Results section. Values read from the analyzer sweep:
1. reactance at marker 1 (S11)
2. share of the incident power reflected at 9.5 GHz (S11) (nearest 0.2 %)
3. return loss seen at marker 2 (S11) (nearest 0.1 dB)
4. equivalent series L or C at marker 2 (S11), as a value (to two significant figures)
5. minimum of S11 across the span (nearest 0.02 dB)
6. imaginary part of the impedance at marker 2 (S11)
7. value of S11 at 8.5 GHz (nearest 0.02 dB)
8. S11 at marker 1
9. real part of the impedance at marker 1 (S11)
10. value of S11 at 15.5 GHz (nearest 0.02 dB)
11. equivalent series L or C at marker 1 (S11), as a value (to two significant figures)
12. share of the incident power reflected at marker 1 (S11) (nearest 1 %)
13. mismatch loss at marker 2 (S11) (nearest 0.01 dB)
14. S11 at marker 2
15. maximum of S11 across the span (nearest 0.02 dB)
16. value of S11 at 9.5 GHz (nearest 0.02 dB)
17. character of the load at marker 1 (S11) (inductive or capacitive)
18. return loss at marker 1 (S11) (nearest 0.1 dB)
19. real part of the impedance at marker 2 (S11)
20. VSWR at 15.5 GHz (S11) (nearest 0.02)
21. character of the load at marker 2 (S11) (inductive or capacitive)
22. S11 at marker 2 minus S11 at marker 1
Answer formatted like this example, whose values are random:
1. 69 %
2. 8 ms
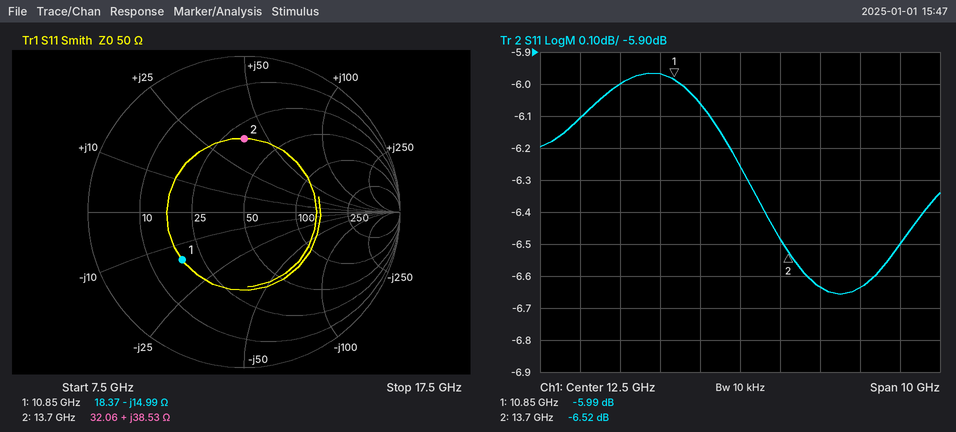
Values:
1. -14.99 Ω
2. 25.2 %
3. 6.6 dB
4. 450 pH
5. -6.66 dB
6. +38.53 Ω
7. -6.10 dB
8. -5.99 dB
9. 18.37 Ω
10. -6.64 dB
11. 980 fF
12. 25 %
13. 1.09 dB
14. -6.52 dB
15. -5.96 dB
16. -6.00 dB
17. capacitive
18. 6.0 dB
19. 32.06 Ω
20. 2.74
21. inductive
22. -0.53 dB
